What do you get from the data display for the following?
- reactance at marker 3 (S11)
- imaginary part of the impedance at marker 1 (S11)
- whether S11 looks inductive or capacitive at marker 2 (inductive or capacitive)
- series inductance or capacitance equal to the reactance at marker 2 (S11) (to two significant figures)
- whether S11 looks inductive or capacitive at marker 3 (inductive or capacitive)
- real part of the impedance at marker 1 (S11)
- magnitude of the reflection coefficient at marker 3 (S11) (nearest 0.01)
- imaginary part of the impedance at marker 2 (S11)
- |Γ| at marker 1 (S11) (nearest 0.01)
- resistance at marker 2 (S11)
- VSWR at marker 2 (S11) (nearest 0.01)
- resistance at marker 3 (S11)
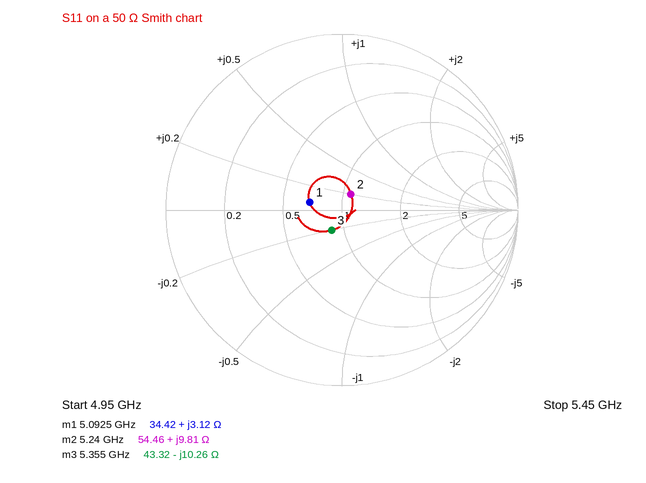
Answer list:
-10.26 Ω
+3.12 Ω
inductive
300 pH
capacitive
34.42 Ω
0.13
+9.81 Ω
0.19
54.46 Ω
1.23
43.32 Ω
